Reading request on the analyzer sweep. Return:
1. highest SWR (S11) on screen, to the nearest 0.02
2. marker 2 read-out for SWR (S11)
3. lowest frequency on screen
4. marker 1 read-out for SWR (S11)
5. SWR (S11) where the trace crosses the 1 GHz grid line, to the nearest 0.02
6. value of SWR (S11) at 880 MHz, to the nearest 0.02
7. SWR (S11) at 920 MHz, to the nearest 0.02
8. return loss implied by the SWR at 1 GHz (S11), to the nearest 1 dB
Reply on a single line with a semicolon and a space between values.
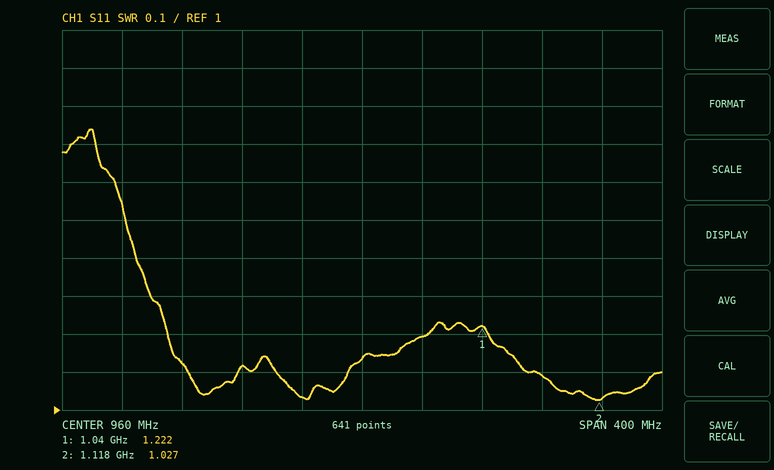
1.74; 1.027; 760 MHz; 1.222; 1.20; 1.12; 1.04; 21 dB
